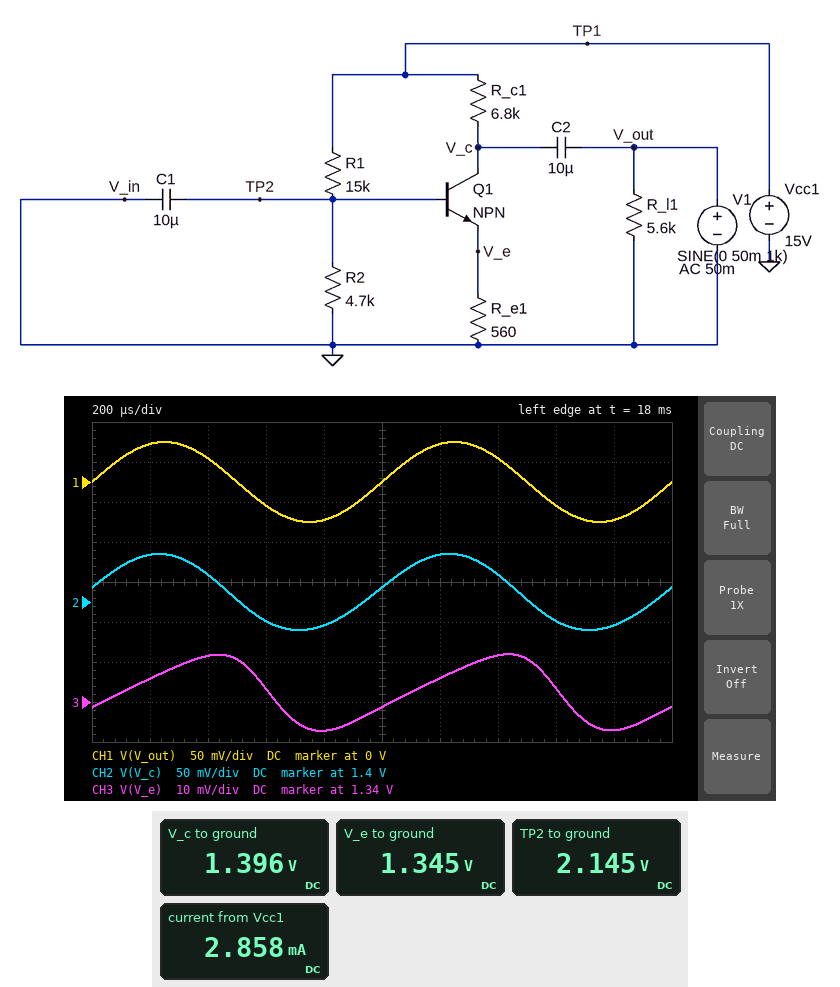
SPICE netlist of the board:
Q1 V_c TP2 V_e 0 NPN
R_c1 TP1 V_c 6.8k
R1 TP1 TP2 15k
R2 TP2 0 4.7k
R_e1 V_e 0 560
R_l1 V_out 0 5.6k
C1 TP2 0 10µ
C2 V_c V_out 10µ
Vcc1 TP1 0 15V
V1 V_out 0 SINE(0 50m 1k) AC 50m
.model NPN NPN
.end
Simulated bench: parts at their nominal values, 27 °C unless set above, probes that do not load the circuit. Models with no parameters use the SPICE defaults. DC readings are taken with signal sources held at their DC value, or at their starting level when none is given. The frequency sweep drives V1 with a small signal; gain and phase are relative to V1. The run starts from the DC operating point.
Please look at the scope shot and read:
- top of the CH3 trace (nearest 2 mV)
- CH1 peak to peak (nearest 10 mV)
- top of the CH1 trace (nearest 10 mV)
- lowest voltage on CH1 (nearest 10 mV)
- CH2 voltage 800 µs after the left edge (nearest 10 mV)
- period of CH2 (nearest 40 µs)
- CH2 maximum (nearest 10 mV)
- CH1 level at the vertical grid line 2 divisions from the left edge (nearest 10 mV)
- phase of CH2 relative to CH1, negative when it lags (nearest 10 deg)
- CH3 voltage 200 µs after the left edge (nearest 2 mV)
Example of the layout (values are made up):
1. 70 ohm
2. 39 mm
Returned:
1. 1.352 V
2. 100 mV
3. 50 mV
4. -50 mV
5. 1.37 V
6. 1.00 ms
7. 1.46 V
8. 30 mV
9. 10 deg
10. 1.346 V
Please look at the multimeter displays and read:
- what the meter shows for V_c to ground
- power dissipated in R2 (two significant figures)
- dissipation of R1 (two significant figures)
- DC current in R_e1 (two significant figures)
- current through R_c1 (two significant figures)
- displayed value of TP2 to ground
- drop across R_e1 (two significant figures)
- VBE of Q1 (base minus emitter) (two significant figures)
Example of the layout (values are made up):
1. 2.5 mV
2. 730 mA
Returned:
1. 1.396 V
2. 980 µW
3. 11 mW
4. 2.4 mA
5. 2.0 mA
6. 2.145 V
7. 1.3 V
8. 800 mV
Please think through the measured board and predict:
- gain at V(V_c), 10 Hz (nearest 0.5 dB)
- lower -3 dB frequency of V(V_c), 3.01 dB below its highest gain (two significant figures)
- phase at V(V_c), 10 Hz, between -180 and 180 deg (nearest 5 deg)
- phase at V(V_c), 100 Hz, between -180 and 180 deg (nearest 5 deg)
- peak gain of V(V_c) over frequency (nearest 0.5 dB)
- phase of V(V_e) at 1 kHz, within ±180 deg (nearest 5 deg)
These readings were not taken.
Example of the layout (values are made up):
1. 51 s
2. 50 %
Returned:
1. -12.0 dB
2. 310 Hz
3. 60 deg
4. 20 deg
5. 0 dB
6. -35 deg
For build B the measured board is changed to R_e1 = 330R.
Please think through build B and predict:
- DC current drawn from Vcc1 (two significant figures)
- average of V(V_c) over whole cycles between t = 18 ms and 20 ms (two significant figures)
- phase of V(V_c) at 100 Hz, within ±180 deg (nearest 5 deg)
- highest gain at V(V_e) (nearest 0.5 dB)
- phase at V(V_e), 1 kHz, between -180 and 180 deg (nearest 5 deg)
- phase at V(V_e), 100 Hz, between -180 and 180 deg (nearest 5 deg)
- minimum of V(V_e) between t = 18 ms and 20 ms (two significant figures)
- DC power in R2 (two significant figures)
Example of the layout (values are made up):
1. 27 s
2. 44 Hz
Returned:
1. 3.0 mA
2. 920 mV
3. 25 deg
4. -6.5 dB
5. -30 deg
6. 10 deg
7. 850 mV
8. 590 µW
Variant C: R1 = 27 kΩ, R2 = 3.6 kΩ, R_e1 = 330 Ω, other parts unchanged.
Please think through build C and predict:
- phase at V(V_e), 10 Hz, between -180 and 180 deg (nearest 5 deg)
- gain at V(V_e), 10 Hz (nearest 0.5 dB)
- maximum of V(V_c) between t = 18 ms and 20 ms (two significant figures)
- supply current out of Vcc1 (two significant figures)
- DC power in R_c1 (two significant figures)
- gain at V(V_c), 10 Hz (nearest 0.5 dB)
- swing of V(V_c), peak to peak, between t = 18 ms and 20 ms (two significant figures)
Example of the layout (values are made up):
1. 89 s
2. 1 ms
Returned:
1. 65 deg
2. -15.5 dB
3. 880 mV
4. 2.6 mA
5. 30 mW
6. -13.5 dB
7. 100 mV
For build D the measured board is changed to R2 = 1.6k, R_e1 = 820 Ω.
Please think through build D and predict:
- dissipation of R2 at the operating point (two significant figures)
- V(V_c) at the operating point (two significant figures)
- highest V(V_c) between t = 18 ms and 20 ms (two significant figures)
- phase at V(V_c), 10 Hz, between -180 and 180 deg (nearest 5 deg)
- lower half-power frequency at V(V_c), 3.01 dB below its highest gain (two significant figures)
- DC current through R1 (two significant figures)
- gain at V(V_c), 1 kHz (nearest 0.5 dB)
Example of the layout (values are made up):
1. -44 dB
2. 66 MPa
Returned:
1. 1.3 mW
2. 9.5 V
3. 9.6 V
4. 15 deg
5. 2.3 Hz
6. 900 µA
7. 0 dB
